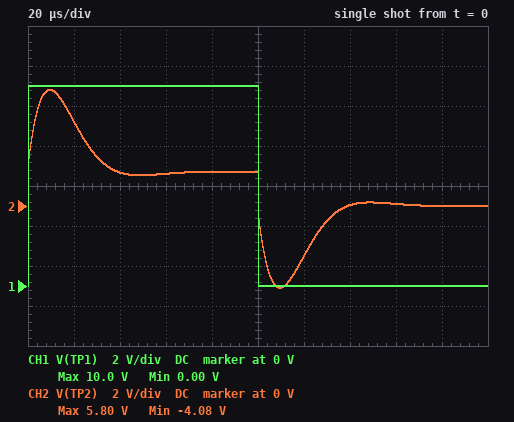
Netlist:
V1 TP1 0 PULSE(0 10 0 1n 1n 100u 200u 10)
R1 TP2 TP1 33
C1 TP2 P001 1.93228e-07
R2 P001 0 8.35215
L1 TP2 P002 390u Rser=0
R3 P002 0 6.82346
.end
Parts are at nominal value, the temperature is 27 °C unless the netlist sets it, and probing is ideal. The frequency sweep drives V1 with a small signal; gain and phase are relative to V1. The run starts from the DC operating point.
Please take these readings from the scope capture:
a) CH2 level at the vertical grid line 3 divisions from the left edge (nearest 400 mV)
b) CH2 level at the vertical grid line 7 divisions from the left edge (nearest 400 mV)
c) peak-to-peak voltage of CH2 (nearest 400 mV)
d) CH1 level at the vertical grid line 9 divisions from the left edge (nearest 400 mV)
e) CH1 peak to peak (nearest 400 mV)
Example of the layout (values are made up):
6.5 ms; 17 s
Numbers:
1.6 V; 0 V; 10.0 V; 0 V; 10.0 V
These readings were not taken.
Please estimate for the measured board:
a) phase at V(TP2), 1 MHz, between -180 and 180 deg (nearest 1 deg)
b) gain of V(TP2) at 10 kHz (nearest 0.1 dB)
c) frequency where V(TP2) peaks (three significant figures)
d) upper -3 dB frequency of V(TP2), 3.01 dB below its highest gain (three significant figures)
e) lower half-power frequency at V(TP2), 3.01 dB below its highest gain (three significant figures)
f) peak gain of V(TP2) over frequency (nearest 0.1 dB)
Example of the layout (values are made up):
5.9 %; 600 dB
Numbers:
-4 deg; -4.2 dB; 18.1 kHz; 36.3 kHz; 9.10 kHz; -1.9 dB
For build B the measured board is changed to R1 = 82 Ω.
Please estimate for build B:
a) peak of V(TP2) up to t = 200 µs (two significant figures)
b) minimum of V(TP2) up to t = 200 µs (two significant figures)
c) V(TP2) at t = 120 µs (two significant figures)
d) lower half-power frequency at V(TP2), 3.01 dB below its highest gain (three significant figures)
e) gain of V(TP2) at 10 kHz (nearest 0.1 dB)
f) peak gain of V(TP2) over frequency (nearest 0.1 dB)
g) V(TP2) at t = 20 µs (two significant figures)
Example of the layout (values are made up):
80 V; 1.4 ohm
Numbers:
3.5 V; -2.7 V; -1.6 V; 12.1 kHz; -9.2 dB; -4.1 dB; 2.4 V
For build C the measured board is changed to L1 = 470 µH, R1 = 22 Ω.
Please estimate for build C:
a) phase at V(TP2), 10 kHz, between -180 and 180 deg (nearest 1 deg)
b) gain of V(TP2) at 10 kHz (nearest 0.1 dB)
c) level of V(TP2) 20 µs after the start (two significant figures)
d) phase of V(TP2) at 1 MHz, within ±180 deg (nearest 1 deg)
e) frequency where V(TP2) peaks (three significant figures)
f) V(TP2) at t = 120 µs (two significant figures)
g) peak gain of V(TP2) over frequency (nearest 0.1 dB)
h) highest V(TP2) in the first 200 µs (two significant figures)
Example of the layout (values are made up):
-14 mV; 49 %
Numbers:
20 deg; -2.1 dB; 5.7 V; -4 deg; 16.4 kHz; -3.3 V; -1.1 dB; 7.1 V
